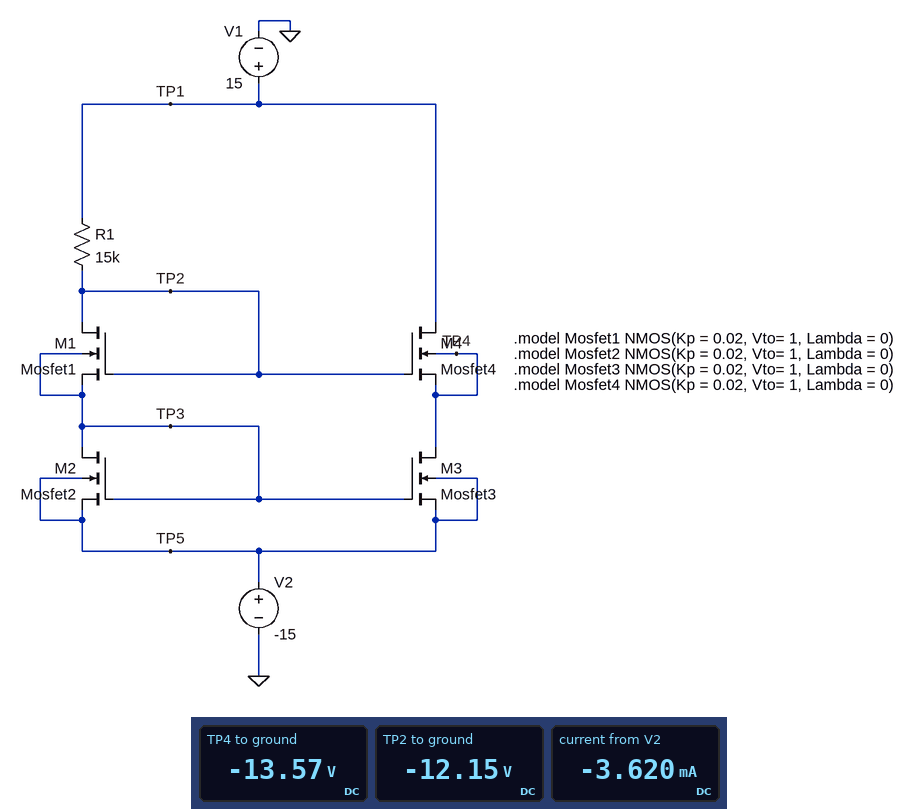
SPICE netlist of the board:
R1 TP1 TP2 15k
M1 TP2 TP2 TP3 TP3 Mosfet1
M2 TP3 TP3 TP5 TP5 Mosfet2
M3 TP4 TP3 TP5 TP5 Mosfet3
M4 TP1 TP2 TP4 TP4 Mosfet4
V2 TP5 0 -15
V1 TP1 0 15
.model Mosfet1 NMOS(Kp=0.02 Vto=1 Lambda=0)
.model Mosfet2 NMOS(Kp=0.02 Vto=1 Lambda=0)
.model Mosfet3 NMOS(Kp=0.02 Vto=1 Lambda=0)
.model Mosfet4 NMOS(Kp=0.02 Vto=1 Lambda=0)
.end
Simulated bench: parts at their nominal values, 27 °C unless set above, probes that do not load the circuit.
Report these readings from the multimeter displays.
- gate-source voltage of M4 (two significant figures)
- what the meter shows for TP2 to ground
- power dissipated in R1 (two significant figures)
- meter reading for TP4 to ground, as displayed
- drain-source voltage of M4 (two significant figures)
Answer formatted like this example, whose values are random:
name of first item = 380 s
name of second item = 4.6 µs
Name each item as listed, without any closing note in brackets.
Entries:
gate-source voltage of M4 = 1.4 V
what the meter shows for TP2 to ground = -12.15 V
power dissipated in R1 = 49 mW
meter reading for TP4 to ground, as displayed = -13.57 V
drain-source voltage of M4 = 29 V
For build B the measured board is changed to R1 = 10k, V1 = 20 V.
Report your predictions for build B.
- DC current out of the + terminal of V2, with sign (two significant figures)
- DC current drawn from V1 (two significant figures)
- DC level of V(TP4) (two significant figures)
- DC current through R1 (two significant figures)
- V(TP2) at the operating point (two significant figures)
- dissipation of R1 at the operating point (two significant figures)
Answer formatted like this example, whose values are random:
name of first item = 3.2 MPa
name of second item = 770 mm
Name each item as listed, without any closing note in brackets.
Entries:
DC current out of the + terminal of V2, with sign = -6.4 mA
DC current drawn from V1 = 6.4 mA
DC level of V(TP4) = -13 V
DC current through R1 = 3.2 mA
V(TP2) at the operating point = -12 V
dissipation of R1 at the operating point = 100 mW
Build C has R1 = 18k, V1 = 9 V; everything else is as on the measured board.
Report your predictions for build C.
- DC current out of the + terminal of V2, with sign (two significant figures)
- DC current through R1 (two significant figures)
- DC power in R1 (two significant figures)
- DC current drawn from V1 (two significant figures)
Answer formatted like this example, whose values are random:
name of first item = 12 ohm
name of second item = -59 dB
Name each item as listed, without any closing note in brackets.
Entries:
DC current out of the + terminal of V2, with sign = -2.4 mA
DC current through R1 = 1.2 mA
DC power in R1 = 25 mW
DC current drawn from V1 = 2.4 mA
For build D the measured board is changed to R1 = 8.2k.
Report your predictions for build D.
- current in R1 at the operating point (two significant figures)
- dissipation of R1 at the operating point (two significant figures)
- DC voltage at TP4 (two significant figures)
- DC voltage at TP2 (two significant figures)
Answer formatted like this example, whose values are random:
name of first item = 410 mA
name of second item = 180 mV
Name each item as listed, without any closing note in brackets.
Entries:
current in R1 at the operating point = 3.3 mA
dissipation of R1 at the operating point = 88 mW
DC voltage at TP4 = -13 V
DC voltage at TP2 = -12 V
